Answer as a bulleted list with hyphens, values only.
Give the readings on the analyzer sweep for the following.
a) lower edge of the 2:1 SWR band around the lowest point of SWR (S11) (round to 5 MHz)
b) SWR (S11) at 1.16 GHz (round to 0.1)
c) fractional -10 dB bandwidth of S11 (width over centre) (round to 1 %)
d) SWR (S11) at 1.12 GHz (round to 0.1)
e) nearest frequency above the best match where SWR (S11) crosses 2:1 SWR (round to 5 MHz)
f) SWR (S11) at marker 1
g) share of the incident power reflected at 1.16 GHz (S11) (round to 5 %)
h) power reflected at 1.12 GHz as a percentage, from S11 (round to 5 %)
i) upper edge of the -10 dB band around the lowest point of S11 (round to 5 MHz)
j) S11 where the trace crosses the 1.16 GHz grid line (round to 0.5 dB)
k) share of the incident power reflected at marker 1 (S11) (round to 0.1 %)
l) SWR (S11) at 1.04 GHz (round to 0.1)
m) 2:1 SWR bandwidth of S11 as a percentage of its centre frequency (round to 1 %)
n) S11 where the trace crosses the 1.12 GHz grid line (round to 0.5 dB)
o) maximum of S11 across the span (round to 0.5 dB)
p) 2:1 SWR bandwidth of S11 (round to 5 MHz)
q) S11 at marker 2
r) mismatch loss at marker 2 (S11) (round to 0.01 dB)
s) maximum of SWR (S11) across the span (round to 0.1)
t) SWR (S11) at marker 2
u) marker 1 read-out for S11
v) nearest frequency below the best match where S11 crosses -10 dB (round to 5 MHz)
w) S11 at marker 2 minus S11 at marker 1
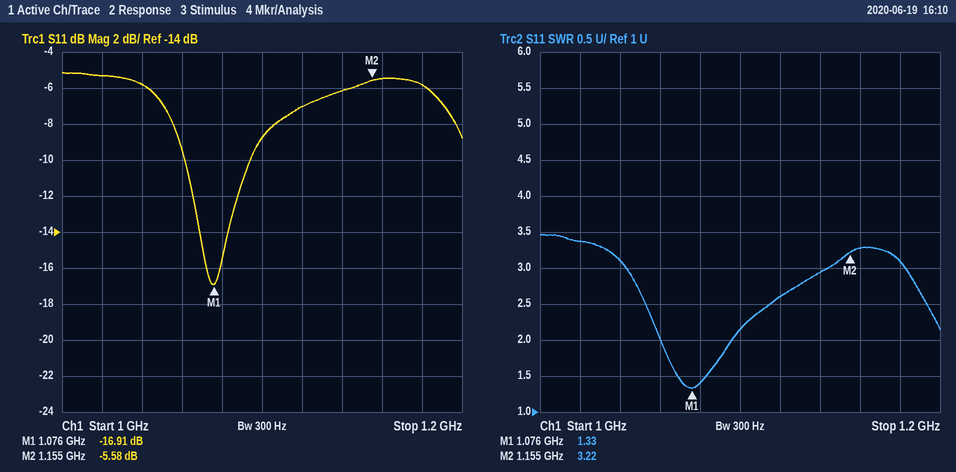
- 1.060 GHz
- 3.3
- 3 %
- 2.6
- 1.095 GHz
- 1.33
- 30 %
- 20 %
- 1.095 GHz
- -5.5 dB
- 2.0 %
- 3.1
- 3 %
- -7.0 dB
- -5.0 dB
- 35 MHz
- -5.58 dB
- 1.41 dB
- 3.5
- 3.22
- -16.91 dB
- 1.060 GHz
- 11.33 dB
